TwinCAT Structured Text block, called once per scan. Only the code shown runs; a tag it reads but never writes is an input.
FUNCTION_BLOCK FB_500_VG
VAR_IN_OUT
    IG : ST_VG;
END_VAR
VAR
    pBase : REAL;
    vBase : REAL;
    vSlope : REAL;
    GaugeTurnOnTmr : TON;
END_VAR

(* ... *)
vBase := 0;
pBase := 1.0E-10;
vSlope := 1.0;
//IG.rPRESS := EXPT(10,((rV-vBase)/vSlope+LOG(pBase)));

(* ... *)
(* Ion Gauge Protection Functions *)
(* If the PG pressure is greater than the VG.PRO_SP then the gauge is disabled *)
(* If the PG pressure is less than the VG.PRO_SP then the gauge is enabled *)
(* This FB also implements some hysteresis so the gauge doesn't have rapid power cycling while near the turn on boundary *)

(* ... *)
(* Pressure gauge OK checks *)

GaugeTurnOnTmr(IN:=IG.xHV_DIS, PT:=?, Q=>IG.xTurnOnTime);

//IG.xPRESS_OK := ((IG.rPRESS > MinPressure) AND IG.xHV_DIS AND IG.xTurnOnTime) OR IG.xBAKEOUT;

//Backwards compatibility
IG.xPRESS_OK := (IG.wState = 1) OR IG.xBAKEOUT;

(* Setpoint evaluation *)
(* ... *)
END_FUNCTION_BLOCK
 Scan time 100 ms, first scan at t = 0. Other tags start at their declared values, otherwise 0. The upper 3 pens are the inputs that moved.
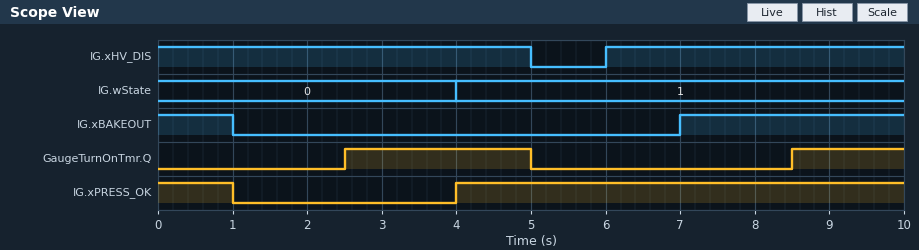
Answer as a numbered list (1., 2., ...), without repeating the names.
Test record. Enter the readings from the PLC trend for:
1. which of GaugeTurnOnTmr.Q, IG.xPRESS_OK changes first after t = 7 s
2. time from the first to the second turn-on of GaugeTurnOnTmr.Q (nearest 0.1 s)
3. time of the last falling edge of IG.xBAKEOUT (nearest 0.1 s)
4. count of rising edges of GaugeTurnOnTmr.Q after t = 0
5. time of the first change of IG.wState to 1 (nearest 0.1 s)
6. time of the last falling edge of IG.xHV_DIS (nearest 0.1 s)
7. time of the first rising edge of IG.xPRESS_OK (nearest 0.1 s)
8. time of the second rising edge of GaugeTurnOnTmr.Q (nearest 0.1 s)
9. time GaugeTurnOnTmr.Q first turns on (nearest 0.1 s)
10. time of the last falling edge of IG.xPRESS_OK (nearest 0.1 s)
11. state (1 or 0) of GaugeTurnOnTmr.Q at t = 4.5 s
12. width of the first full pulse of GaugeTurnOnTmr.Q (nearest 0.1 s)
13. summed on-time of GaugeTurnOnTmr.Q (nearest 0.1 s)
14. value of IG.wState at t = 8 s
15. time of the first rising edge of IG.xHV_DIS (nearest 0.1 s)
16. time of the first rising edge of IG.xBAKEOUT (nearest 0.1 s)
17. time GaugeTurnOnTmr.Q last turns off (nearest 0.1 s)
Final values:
1. GaugeTurnOnTmr.Q
2. 6.0 s
3. 1.0 s
4. 2
5. 4.0 s
6. 5.0 s
7. 4.0 s
8. 8.5 s
9. 2.5 s
10. 1.0 s
11. 1
12. 2.5 s
13. 4.0 s
14. 1
15. 6.0 s
16. 7.0 s
17. 5.0 s
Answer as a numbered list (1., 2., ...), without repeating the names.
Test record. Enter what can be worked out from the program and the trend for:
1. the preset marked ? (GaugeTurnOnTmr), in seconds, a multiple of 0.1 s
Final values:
1. 2.5 s
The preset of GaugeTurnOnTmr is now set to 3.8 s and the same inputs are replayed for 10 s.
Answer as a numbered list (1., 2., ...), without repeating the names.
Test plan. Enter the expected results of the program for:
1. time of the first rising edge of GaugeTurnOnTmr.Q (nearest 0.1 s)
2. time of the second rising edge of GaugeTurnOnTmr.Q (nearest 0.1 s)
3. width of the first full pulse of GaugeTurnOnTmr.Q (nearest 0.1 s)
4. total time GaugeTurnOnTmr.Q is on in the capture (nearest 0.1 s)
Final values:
1. 3.8 s
2. 9.8 s
3. 1.2 s
4. 1.4 s
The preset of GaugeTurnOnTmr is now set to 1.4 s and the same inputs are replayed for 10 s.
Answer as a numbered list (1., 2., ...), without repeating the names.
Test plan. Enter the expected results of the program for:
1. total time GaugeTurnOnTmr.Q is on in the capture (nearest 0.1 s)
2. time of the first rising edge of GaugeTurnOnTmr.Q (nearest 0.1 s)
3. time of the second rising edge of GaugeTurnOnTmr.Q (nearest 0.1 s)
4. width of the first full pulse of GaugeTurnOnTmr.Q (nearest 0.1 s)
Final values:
1. 6.2 s
2. 1.4 s
3. 7.4 s
4. 3.6 s
